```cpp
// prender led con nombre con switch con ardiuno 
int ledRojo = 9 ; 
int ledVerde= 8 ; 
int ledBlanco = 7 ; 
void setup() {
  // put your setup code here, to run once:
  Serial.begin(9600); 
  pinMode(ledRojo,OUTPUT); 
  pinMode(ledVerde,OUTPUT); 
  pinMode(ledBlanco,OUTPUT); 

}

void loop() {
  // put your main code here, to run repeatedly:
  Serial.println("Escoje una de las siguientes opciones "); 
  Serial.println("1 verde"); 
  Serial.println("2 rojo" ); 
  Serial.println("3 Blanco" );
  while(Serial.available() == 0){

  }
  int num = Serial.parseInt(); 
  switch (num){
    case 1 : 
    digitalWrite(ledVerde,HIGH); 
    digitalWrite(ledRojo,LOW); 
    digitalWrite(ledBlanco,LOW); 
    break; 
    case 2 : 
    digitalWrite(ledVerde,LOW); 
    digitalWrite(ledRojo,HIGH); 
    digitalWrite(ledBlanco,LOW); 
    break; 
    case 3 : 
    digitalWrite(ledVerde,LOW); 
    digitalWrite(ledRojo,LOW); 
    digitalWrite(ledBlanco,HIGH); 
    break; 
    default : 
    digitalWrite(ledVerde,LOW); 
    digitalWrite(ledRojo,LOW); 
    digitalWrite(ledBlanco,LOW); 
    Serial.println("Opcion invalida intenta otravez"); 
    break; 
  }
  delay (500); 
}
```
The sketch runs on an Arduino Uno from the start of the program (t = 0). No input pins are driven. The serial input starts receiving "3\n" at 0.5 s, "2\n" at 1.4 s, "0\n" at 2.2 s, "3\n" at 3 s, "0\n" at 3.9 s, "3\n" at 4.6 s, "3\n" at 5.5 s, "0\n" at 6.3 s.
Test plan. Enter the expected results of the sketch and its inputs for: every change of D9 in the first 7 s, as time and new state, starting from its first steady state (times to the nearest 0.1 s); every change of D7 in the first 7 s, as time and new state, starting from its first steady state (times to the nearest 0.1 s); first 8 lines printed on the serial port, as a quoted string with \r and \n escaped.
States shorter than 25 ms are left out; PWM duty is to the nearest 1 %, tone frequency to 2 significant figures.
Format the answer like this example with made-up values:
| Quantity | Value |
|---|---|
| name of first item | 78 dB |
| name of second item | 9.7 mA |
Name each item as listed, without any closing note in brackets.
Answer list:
| Quantity | Value |
|---|---|
| every change of D9 in the first 7 s, as time and new state, starting from its first steady state | 0 s low; 1.4 s high; 2.2 s low |
| every change of D7 in the first 7 s, as time and new state, starting from its first steady state | 0 s low; 0.5 s high; 1.4 s low; 3 s high; 3.9 s low; 4.6 s high; 6.3 s low |
| first 8 lines printed on the serial port, as a quoted string with \r and \n escaped | "Escoje una de las siguientes opciones \r\n1 verde\r\n2 rojo\r\n3 Blanco\r\nEscoje una de las siguientes opciones \r\n1 verde\r\n2 rojo\r\n3 Blanco\r\n" |
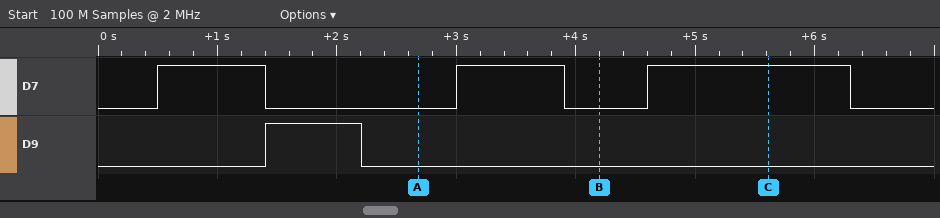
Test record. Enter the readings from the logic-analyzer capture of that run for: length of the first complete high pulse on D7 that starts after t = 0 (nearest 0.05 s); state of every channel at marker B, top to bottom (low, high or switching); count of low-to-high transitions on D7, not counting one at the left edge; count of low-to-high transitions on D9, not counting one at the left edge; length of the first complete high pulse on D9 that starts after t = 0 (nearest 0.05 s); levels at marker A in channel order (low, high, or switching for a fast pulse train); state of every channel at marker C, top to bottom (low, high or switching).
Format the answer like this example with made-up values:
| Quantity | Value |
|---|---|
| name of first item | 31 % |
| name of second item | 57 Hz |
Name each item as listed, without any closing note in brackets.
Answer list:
| Quantity | Value |
|---|---|
| length of the first complete high pulse on D7 that starts after t = 0 | 0.90 s |
| state of every channel at marker B, top to bottom | D7 low, D9 low |
| count of low-to-high transitions on D7, not counting one at the left edge | 3 |
| count of low-to-high transitions on D9, not counting one at the left edge | 1 |
| length of the first complete high pulse on D9 that starts after t = 0 | 0.80 s |
| levels at marker A in channel order | D7 low, D9 low |
| state of every channel at marker C, top to bottom | D7 high, D9 low |
